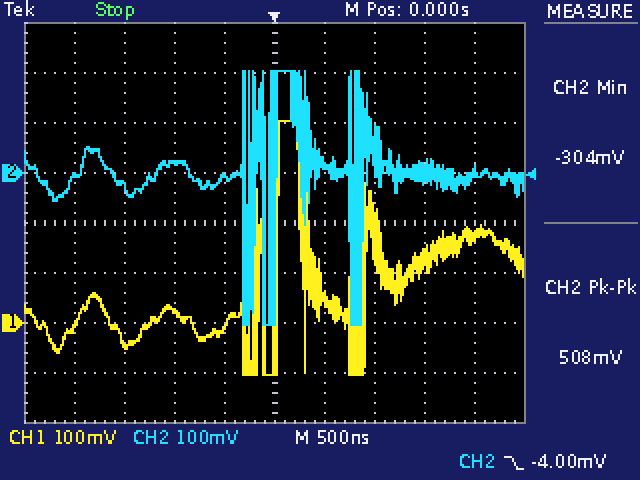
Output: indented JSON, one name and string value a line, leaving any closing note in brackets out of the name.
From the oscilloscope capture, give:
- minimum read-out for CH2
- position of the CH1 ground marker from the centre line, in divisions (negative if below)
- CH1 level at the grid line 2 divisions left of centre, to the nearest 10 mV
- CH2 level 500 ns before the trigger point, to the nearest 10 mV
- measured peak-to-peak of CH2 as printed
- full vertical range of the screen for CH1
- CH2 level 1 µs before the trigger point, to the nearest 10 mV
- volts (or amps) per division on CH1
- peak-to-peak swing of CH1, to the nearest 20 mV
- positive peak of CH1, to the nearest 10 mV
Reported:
{
  "minimum read-out for CH2": "-304 mV",
  "position of the CH1 ground marker from the centre line, in divisions": "-2.0 div",
  "CH1 level at the grid line 2 divisions left of centre, to the nearest 10 mV": "20 mV",
  "CH2 level 500 ns before the trigger point, to the nearest 10 mV": "-10 mV",
  "measured peak-to-peak of CH2 as printed": "508 mV",
  "full vertical range of the screen for CH1": "800 mV",
  "CH2 level 1 µs before the trigger point, to the nearest 10 mV": "20 mV",
  "volts (or amps) per division on CH1": "100 mV",
  "peak-to-peak swing of CH1, to the nearest 20 mV": "500 mV",
  "positive peak of CH1, to the nearest 10 mV": "400 mV"
}
